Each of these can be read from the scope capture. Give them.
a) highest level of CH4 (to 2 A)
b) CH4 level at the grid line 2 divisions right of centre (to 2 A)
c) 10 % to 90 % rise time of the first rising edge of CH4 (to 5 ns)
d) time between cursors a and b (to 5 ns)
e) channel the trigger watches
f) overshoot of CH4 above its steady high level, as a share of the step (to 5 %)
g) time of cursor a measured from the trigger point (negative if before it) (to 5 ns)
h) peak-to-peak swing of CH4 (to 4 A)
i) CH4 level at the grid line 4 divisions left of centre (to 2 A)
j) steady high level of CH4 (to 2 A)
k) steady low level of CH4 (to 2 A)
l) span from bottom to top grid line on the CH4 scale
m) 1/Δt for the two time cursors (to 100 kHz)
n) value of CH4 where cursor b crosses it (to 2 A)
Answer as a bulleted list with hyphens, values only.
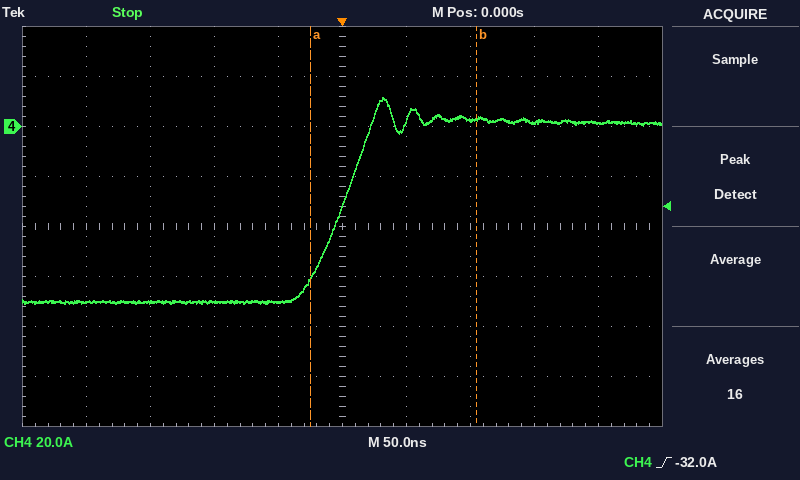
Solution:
- 12 A
- 2 A
- 45 ns
- 130 ns
- CH4
- 15 %
- -25 ns
- 84 A
- -70 A
- 2 A
- -70 A
- 160 A
- 7.7 MHz
- 4 A
